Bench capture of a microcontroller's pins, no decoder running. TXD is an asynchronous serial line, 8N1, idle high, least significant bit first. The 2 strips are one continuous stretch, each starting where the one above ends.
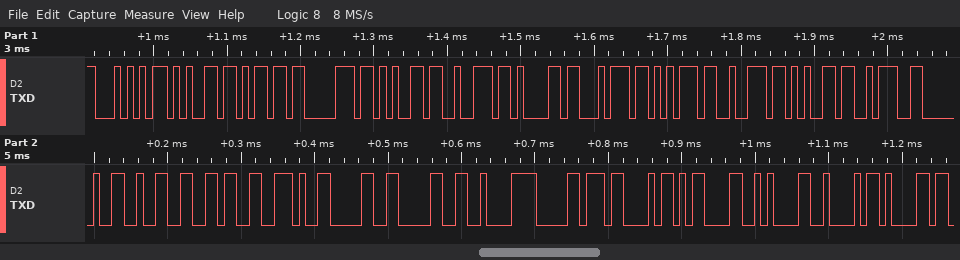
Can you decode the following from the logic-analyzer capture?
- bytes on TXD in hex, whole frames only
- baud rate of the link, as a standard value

54 65 6D 70 65 72 61 74 75 72 65 3A 20 32 36 2E 30 30 C2 B0 43 0D 0A 42 61
115200 baud
